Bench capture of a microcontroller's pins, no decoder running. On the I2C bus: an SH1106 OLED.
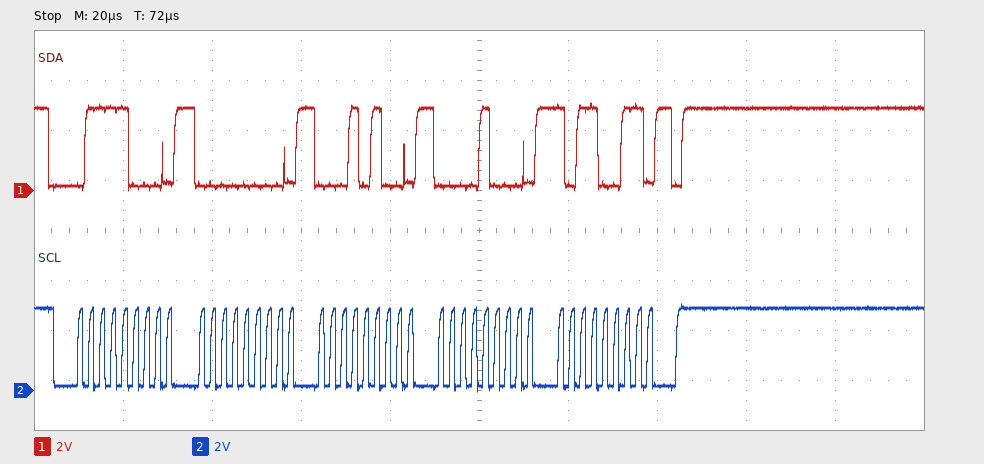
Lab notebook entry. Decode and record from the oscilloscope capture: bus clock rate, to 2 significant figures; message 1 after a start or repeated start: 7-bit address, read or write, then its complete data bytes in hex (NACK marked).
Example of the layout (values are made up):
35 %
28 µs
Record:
400 kHz
0x3C write: 00 14 08 B3
